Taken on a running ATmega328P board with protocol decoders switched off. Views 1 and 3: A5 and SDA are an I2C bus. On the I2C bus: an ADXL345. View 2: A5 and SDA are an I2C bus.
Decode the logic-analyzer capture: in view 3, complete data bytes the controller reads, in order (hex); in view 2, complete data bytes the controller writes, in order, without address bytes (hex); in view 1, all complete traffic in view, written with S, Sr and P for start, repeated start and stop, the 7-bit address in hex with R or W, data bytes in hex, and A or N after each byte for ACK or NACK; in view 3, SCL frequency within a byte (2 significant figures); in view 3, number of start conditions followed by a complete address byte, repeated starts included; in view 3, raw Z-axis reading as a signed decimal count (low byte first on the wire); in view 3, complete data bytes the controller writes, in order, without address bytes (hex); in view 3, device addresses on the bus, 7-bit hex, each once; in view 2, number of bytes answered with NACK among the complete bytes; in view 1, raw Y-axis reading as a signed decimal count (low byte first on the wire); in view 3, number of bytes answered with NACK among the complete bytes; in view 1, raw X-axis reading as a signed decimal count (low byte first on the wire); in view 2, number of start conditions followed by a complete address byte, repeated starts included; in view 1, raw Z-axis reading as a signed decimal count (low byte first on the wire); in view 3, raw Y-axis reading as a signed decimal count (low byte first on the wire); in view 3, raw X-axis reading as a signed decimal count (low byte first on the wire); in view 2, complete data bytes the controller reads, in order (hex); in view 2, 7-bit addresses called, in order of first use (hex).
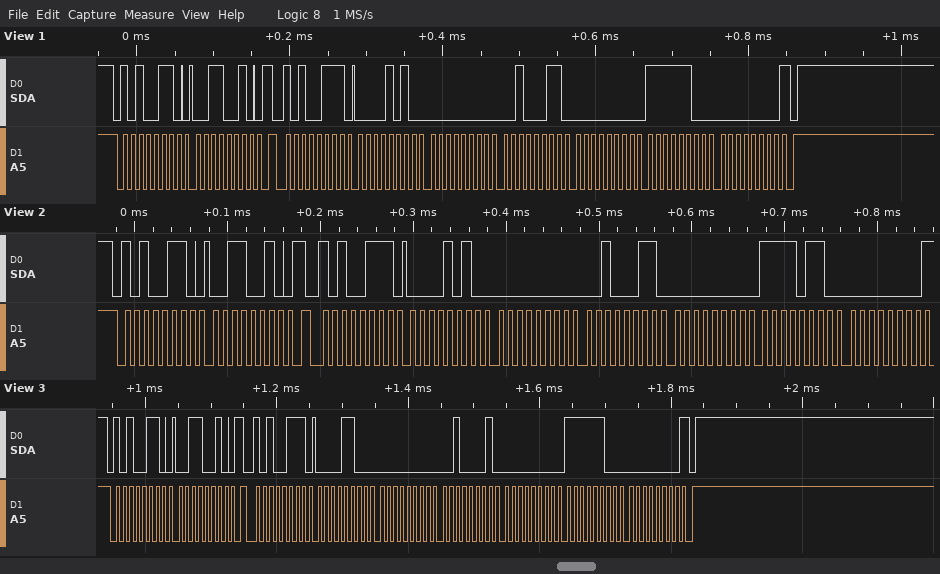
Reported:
0C 00 21 00 FC 00
32
S 53W A 32 A Sr 53R A 0A A 00 A 23 A 00 A FC A 00 N P
100 kHz
2
252
32
0x53
1
35
1
10
2
252
33
12
0A 00 23 00 F6 00
0x53
